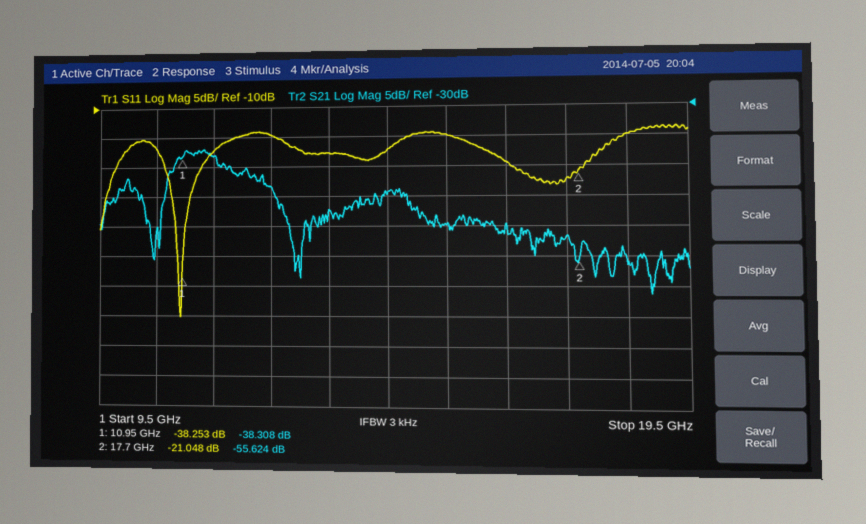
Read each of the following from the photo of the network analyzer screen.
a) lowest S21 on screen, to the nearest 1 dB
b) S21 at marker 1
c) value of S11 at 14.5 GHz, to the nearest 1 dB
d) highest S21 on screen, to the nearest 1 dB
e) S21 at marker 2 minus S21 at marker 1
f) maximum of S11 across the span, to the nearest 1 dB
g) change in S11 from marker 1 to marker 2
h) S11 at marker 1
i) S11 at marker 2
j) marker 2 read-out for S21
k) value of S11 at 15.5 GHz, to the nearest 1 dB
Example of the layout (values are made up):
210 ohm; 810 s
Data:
-61 dB; -38.308 dB; -17 dB; -37 dB; -17.316 dB; -14 dB; 17.205 dB; -38.253 dB; -21.048 dB; -55.624 dB; -15 dB
